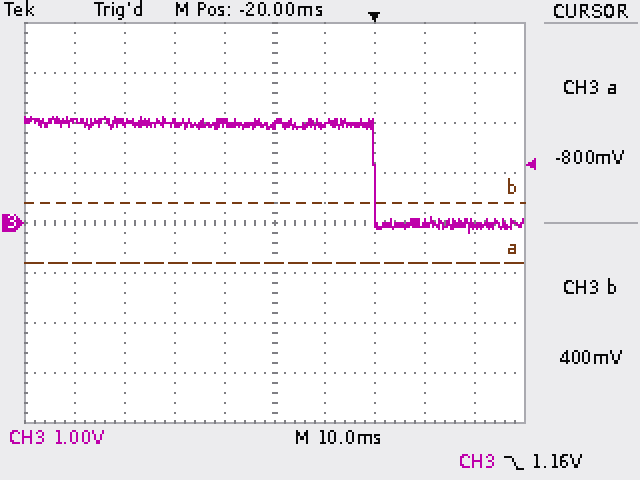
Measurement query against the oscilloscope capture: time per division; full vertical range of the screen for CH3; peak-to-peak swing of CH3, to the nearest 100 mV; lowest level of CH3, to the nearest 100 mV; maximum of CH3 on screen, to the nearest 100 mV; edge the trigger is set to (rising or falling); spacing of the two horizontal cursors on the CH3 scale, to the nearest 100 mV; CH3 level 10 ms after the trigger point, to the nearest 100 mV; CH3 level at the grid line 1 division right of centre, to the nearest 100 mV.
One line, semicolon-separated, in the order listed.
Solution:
10 ms; 8 V; 2.3 V; -200 mV; 2.1 V; falling; 1.2 V; 0.0 V; 1.9 V
